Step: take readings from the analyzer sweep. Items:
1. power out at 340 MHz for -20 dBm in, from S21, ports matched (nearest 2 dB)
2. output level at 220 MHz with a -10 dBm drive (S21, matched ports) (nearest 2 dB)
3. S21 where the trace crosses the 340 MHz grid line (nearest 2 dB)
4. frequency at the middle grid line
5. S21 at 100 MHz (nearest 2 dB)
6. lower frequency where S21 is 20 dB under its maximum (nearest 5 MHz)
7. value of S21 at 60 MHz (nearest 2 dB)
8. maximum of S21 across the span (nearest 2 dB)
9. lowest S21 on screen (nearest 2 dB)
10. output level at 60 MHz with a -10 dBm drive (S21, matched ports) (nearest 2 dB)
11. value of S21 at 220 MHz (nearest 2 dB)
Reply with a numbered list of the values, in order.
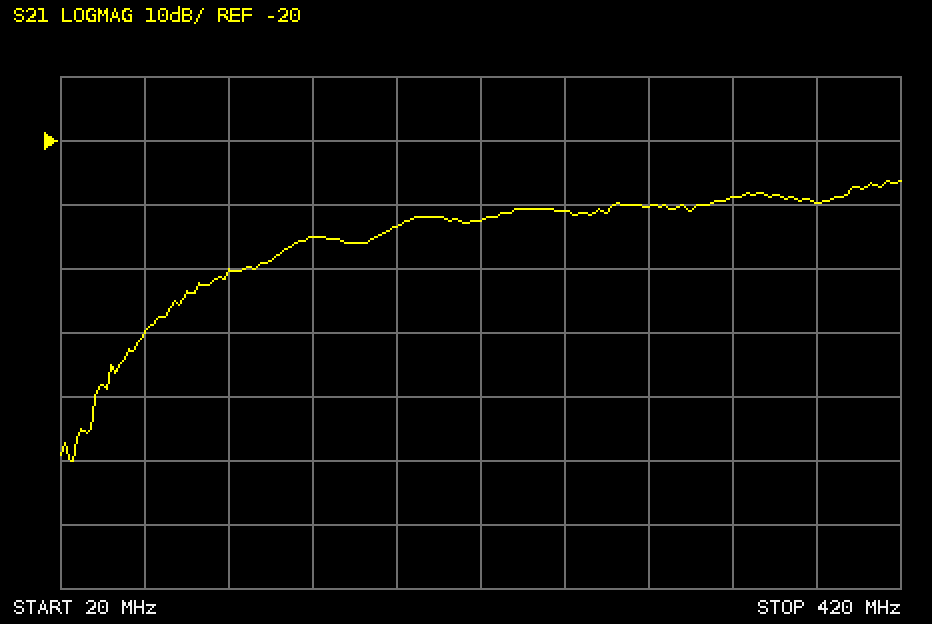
1. -48 dBm
2. -42 dBm
3. -28 dB
4. 220 MHz
5. -40 dB
6. 70 MHz
7. -50 dB
8. -26 dB
9. -70 dB
10. -60 dBm
11. -32 dB
